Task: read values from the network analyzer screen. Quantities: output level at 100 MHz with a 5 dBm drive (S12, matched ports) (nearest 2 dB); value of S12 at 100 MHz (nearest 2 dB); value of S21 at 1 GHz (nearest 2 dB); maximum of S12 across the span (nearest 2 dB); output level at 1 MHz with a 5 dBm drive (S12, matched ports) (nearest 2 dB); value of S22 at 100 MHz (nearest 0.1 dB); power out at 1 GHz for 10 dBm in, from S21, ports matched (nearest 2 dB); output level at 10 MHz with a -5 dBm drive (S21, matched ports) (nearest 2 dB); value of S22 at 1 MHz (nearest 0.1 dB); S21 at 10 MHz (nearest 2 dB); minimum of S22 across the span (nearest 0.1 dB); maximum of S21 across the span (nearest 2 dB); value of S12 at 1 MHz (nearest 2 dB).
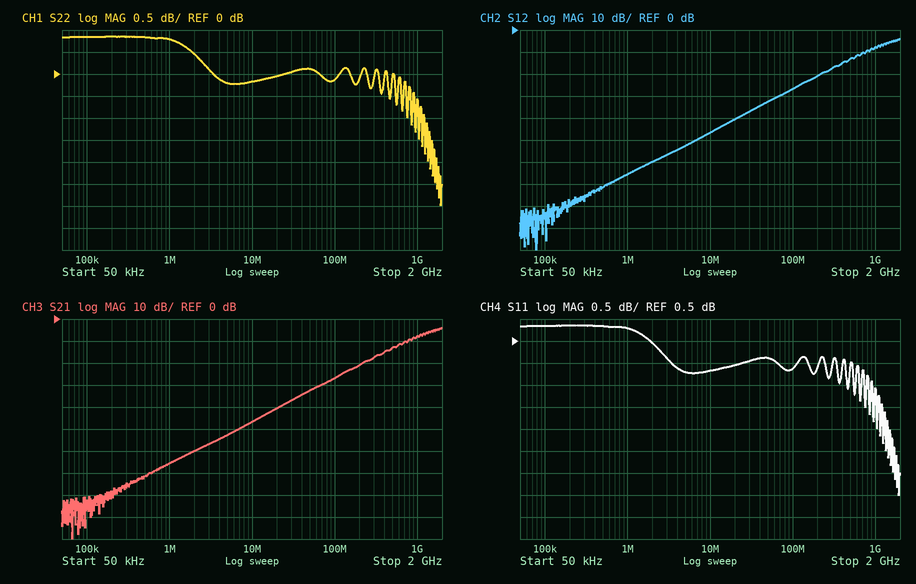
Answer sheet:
-22 dBm
-26 dB
-8 dB
-4 dB
-60 dBm
-0.1 dB
2 dBm
-52 dBm
0.8 dB
-46 dB
-3.0 dB
-4 dB
-66 dB
